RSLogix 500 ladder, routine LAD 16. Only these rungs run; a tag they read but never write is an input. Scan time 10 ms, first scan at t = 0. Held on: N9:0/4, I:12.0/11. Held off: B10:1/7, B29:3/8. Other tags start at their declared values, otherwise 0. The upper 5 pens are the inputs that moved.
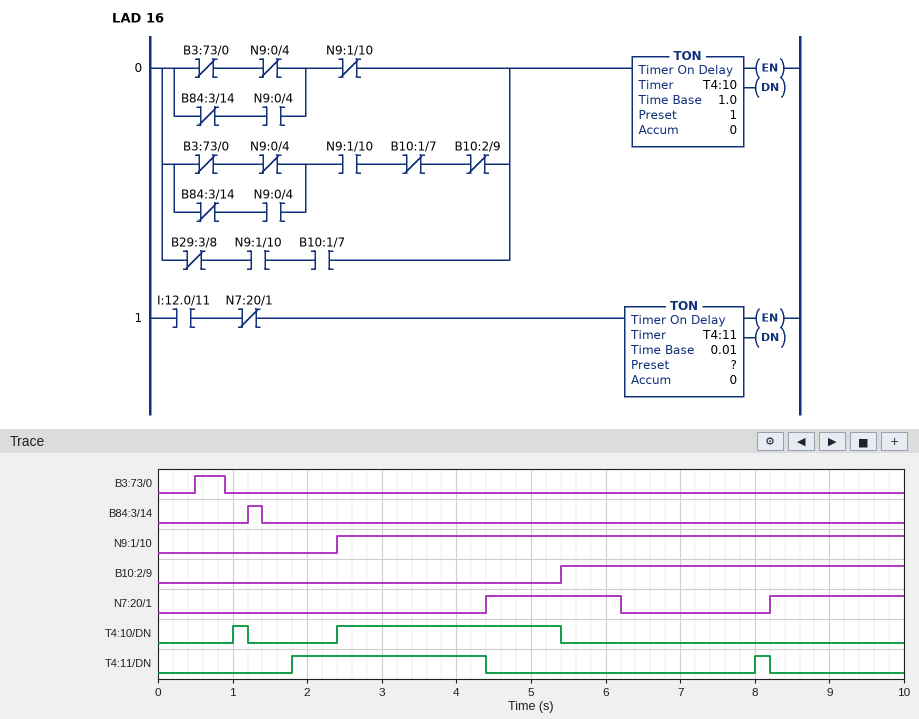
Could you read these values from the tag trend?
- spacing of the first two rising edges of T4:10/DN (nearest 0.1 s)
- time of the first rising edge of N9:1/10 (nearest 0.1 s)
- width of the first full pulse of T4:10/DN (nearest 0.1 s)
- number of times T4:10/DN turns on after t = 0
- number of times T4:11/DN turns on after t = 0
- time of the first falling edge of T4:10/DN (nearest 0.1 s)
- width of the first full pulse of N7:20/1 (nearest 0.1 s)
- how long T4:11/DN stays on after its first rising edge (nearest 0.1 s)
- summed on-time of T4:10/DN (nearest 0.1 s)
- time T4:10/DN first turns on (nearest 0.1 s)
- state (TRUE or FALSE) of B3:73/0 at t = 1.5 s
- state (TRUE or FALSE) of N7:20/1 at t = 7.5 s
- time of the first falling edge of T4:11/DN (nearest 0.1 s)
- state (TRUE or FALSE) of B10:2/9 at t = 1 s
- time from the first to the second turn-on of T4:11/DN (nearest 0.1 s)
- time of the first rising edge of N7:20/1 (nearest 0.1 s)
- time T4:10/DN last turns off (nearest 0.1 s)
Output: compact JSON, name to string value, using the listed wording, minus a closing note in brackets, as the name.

{"spacing of the first two rising edges of T4:10/DN": "1.4 s", "time of the first rising edge of N9:1/10": "2.4 s", "width of the first full pulse of T4:10/DN": "0.2 s", "number of times T4:10/DN turns on after t = 0": "2", "number of times T4:11/DN turns on after t = 0": "2", "time of the first falling edge of T4:10/DN": "1.2 s", "width of the first full pulse of N7:20/1": "1.8 s", "how long T4:11/DN stays on after its first rising edge": "2.6 s", "summed on-time of T4:10/DN": "3.2 s", "time T4:10/DN first turns on": "1.0 s", "state (TRUE or FALSE) of B3:73/0 at t = 1.5 s": "FALSE", "state (TRUE or FALSE) of N7:20/1 at t = 7.5 s": "FALSE", "time of the first falling edge of T4:11/DN": "4.4 s", "state (TRUE or FALSE) of B10:2/9 at t = 1 s": "FALSE", "time from the first to the second turn-on of T4:11/DN": "6.2 s", "time of the first rising edge of N7:20/1": "4.4 s", "time T4:10/DN last turns off": "5.4 s"}
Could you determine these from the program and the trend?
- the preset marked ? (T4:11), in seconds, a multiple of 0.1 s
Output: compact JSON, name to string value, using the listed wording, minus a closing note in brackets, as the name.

{"the preset marked ? (T4:11), in seconds, a multiple of 0.1 s": "1.8 s"}
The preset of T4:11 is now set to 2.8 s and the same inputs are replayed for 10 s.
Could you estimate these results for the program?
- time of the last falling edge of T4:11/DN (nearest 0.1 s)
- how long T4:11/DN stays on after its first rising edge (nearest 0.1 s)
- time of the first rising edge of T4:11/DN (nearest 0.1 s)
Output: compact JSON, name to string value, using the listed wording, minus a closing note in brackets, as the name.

{"time of the last falling edge of T4:11/DN": "4.4 s", "how long T4:11/DN stays on after its first rising edge": "1.6 s", "time of the first rising edge of T4:11/DN": "2.8 s"}
